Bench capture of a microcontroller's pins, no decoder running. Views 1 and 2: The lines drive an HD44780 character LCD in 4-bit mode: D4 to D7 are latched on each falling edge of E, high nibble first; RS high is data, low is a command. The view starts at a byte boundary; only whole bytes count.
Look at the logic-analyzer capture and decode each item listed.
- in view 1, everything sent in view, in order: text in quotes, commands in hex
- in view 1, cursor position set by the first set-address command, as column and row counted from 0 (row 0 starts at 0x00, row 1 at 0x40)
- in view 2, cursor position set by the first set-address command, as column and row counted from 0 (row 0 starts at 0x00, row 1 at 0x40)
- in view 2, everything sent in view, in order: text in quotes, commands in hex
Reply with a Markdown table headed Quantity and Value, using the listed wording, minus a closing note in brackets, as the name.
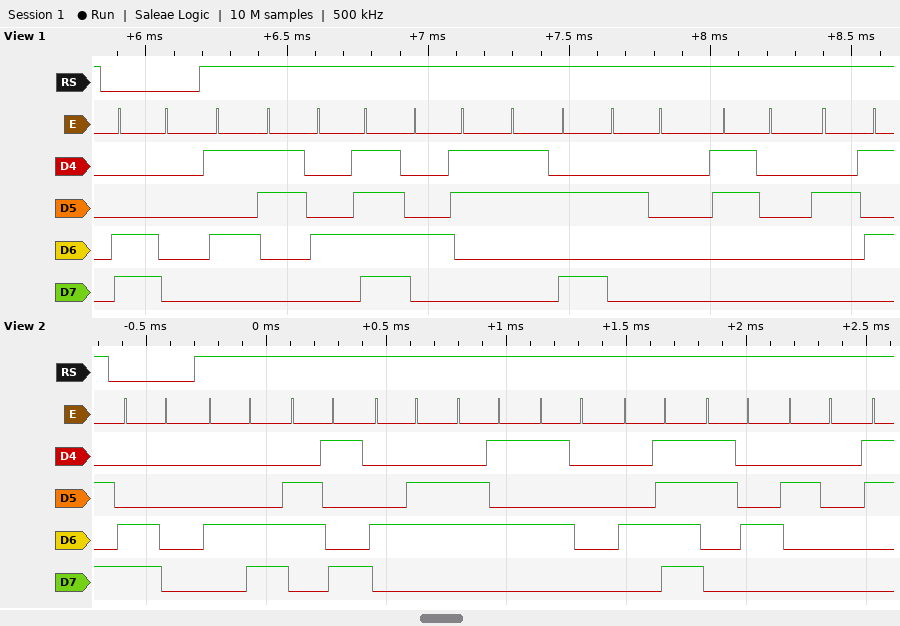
| Quantity | Value |
|---|---|
| in view 1, everything sent in view, in order: text in quotes, commands in hex | 0xC0 "SOC: 0%" |
| in view 1, cursor position set by the first set-address command, as column and row counted from 0 | column 0, row 1 |
| in view 2, cursor position set by the first set-address command, as column and row counted from 0 | column 0, row 1 |
| in view 2, everything sent in view, in order: text in quotes, commands in hex | 0xC0 "LiFePO4 " |
